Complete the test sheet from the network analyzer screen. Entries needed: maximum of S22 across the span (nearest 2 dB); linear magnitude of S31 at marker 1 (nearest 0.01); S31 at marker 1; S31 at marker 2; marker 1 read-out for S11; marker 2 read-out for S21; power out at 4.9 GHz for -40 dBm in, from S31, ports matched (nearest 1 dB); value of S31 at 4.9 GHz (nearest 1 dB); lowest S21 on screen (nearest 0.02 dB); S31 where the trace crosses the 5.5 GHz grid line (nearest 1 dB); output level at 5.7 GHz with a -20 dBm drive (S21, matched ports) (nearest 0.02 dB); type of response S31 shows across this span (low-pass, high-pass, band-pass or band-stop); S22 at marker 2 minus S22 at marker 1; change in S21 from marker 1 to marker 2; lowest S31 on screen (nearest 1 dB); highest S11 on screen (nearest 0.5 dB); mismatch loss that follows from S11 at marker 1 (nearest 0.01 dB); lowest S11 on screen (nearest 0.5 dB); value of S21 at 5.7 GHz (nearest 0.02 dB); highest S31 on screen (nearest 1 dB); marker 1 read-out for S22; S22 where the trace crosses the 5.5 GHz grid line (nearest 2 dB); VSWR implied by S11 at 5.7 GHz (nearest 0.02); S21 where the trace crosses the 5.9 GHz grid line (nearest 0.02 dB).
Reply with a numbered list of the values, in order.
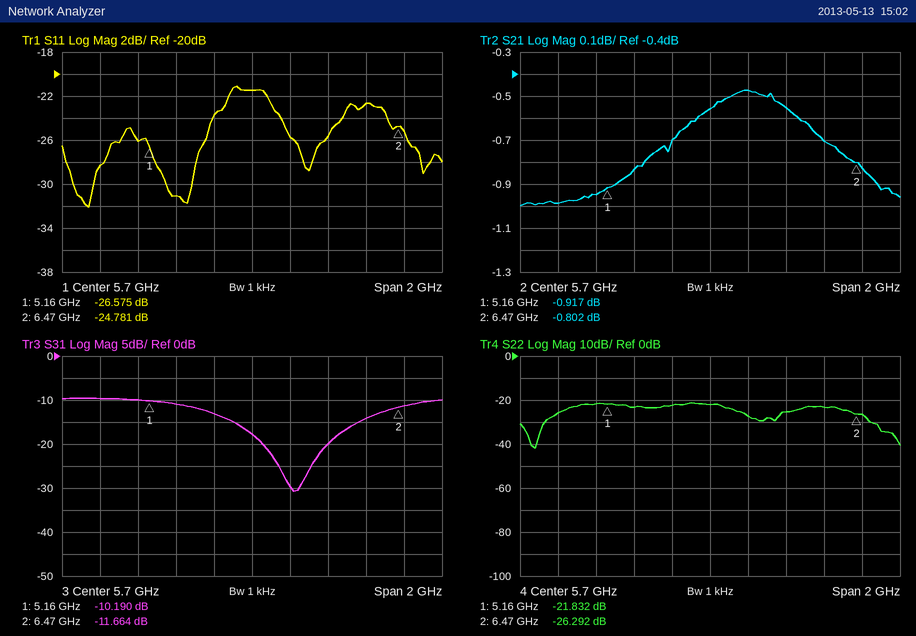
1. -22 dB
2. 0.31
3. -10.190 dB
4. -11.664 dB
5. -26.575 dB
6. -0.802 dB
7. -50 dBm
8. -10 dB
9. -1.00 dB
10. -13 dB
11. -20.56 dBm
12. band-stop
13. -4.460 dB
14. 0.115 dB
15. -31 dB
16. -21.0 dB
17. 0.01 dB
18. -32.0 dB
19. -0.56 dB
20. -10 dB
21. -21.832 dB
22. -22 dB
23. 1.18
24. -0.48 dB
